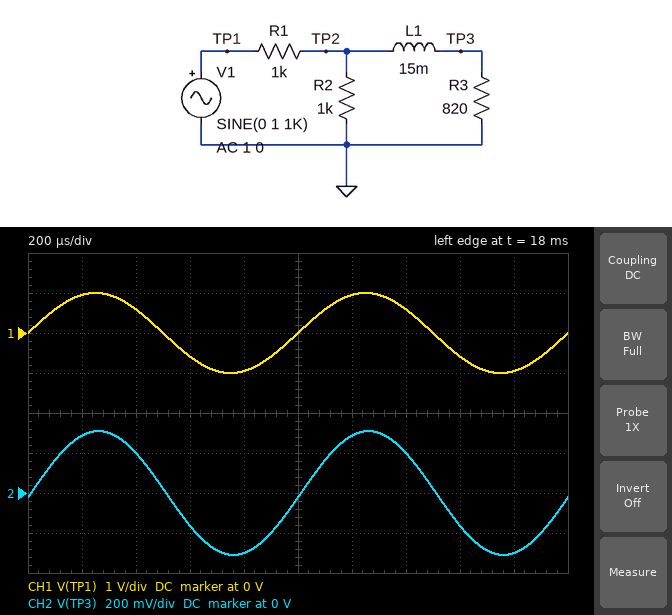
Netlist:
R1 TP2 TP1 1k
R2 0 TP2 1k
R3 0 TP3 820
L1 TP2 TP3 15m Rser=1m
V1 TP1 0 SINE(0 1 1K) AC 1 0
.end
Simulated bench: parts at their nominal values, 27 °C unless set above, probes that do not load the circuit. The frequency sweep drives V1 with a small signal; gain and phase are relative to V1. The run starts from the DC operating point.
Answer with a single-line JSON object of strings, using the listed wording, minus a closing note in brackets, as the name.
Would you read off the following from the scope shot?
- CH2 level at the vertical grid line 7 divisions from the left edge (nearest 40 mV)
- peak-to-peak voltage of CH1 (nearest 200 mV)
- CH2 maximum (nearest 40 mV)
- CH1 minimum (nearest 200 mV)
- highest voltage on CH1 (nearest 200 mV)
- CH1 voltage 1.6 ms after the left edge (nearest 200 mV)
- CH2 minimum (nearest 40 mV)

{"CH2 level at the vertical grid line 7 divisions from the left edge": "200 mV", "peak-to-peak voltage of CH1": "2.0 V", "CH2 maximum": "320 mV", "CH1 minimum": "-1.0 V", "highest voltage on CH1": "1.0 V", "CH1 voltage 1.6 ms after the left edge": "-600 mV", "CH2 minimum": "-320 mV"}
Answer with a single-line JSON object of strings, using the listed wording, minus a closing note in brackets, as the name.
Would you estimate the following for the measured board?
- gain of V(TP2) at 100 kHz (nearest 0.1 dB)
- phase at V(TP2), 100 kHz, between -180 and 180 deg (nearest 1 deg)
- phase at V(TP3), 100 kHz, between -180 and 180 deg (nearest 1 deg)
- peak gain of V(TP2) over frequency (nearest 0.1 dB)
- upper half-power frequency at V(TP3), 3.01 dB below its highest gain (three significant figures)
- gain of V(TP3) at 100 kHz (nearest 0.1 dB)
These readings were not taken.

{"gain of V(TP2) at 100 kHz": "-6.1 dB", "phase at V(TP2), 100 kHz, between -180 and 180 deg": "3 deg", "phase at V(TP3), 100 kHz, between -180 and 180 deg": "-82 deg", "peak gain of V(TP2) over frequency": "-6.0 dB", "upper half-power frequency at V(TP3), 3.01 dB below its highest gain": "14.0 kHz", "gain of V(TP3) at 100 kHz": "-27.3 dB"}
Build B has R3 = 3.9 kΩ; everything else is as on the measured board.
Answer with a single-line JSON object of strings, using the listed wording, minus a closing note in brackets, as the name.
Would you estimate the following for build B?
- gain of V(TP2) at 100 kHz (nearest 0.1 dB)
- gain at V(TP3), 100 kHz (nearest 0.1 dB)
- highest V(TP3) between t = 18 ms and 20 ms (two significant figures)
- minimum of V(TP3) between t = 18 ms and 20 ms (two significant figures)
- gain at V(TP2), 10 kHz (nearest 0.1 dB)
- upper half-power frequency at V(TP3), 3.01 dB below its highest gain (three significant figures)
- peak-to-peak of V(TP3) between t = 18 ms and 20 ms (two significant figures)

{"gain of V(TP2) at 100 kHz": "-6.2 dB", "gain at V(TP3), 100 kHz": "-14.5 dB", "highest V(TP3) between t = 18 ms and 20 ms": "440 mV", "minimum of V(TP3) between t = 18 ms and 20 ms": "-440 mV", "gain at V(TP2), 10 kHz": "-7.0 dB", "upper half-power frequency at V(TP3), 3.01 dB below its highest gain": "46.7 kHz", "peak-to-peak of V(TP3) between t = 18 ms and 20 ms": "890 mV"}
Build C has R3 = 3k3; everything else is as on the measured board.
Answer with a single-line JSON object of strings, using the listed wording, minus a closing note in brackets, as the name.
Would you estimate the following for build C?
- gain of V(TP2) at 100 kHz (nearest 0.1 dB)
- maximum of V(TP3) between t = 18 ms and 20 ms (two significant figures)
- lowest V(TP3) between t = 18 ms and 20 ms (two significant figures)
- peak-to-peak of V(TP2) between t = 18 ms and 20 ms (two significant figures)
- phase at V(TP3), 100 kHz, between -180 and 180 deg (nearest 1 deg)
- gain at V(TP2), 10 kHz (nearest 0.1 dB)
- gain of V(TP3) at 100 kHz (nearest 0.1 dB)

{"gain of V(TP2) at 100 kHz": "-6.2 dB", "maximum of V(TP3) between t = 18 ms and 20 ms": "430 mV", "lowest V(TP3) between t = 18 ms and 20 ms": "-430 mV", "peak-to-peak of V(TP2) between t = 18 ms and 20 ms": "870 mV", "phase at V(TP3), 100 kHz, between -180 and 180 deg": "-68 deg", "gain at V(TP2), 10 kHz": "-7.2 dB", "gain of V(TP3) at 100 kHz": "-15.8 dB"}
